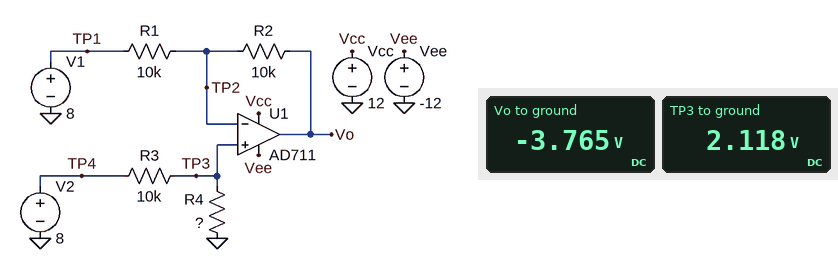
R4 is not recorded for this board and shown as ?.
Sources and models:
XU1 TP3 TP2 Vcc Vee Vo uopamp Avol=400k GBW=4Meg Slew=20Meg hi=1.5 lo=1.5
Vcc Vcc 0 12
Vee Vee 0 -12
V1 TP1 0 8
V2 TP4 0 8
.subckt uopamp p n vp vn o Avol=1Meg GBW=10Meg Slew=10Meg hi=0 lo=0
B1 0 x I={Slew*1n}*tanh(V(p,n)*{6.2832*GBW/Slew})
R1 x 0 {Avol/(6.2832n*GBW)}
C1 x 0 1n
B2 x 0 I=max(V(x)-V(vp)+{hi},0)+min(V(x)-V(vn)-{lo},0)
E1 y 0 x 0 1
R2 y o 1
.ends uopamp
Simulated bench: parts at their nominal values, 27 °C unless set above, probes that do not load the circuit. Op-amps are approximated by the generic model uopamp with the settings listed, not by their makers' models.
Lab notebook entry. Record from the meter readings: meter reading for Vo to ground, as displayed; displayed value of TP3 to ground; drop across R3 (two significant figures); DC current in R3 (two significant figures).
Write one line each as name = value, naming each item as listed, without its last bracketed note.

meter reading for Vo to ground, as displayed = -3.765 V
displayed value of TP3 to ground = 2.118 V
drop across R3 = 5.9 V
DC current in R3 = 590 µA
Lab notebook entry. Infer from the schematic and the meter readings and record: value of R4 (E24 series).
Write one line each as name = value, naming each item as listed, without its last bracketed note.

value of R4 = 3.6 kΩ
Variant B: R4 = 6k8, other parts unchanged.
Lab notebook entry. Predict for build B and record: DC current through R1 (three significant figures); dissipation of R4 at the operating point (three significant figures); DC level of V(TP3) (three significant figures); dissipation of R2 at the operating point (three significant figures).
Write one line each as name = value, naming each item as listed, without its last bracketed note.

DC current through R1 = 476 µA
dissipation of R4 at the operating point = 1.54 mW
DC level of V(TP3) = 3.24 V
dissipation of R2 at the operating point = 2.27 mW
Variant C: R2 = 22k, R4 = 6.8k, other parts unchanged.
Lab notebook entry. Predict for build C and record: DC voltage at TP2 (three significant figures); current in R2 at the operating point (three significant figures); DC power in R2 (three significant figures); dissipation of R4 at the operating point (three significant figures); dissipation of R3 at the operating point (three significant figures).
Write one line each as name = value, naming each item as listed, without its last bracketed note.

DC voltage at TP2 = 3.24 V
current in R2 at the operating point = 476 µA
DC power in R2 = 4.99 mW
dissipation of R4 at the operating point = 1.54 mW
dissipation of R3 at the operating point = 2.27 mW
